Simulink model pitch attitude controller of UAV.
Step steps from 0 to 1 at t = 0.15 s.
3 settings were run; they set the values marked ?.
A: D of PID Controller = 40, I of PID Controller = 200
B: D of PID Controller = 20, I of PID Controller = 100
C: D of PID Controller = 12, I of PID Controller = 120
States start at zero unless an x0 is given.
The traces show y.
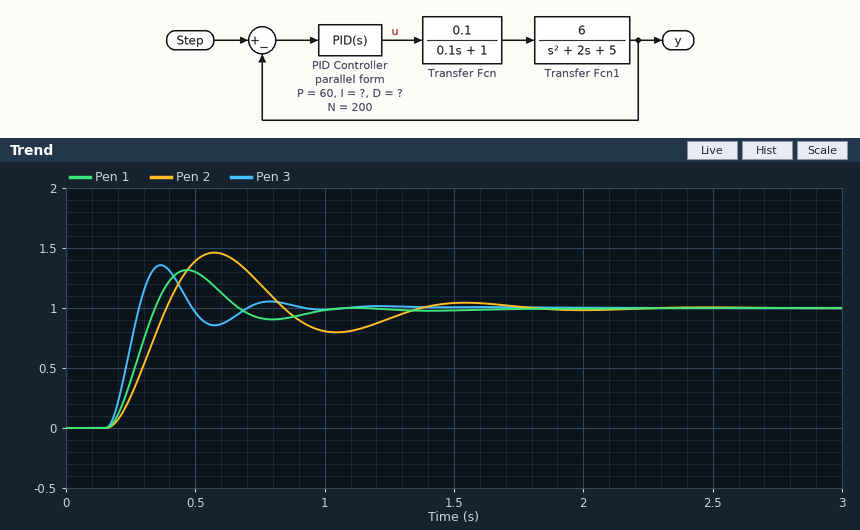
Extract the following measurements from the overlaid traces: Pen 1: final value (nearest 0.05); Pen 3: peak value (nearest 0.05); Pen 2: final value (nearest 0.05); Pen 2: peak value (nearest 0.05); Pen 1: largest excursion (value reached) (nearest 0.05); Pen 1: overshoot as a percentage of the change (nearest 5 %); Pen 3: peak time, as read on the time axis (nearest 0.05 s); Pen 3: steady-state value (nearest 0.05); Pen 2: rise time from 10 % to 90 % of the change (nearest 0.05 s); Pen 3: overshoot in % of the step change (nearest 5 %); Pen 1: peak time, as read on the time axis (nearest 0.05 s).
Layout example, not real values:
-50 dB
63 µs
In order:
1.00
1.35
1.00
1.45
1.30
30 %
0.35 s
1.00
0.15 s
35 %
0.45 s
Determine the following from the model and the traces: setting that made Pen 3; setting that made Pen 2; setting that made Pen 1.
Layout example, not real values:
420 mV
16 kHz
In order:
A
C
B
